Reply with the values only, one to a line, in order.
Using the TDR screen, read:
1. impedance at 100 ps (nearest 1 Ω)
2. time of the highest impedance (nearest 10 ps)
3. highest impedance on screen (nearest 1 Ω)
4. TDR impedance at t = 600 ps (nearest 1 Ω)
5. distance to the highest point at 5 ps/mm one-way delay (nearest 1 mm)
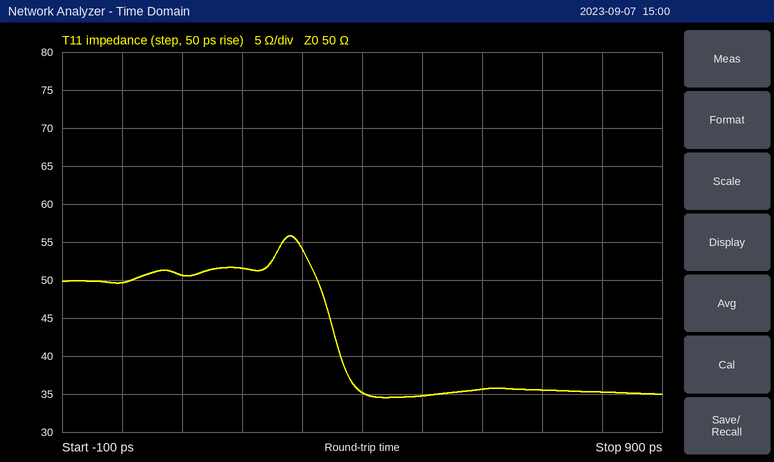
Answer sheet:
51 Ω
280 ps
56 Ω
36 Ω
28 mm
